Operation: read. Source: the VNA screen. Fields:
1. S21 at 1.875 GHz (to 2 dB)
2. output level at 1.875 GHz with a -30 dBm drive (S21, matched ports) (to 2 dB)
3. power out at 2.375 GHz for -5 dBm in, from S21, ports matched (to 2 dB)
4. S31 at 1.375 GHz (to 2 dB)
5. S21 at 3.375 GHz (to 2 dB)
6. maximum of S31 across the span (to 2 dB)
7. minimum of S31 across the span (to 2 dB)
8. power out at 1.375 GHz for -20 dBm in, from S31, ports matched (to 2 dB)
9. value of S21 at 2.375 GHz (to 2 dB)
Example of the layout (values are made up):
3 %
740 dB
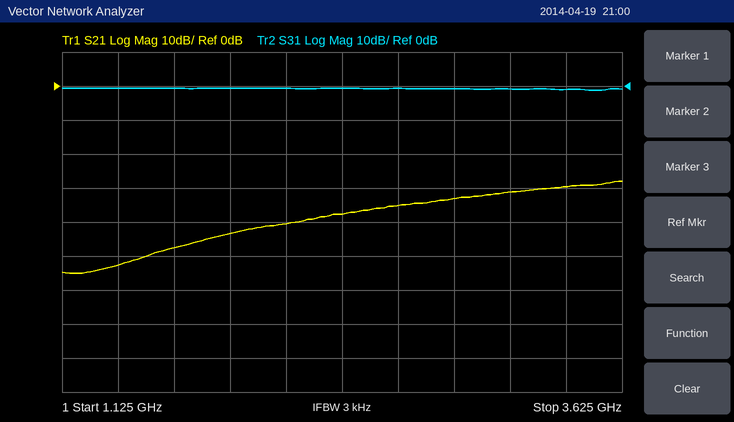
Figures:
-44 dB
-74 dBm
-42 dBm
0 dB
-30 dB
0 dB
-2 dB
-20 dBm
-38 dB
